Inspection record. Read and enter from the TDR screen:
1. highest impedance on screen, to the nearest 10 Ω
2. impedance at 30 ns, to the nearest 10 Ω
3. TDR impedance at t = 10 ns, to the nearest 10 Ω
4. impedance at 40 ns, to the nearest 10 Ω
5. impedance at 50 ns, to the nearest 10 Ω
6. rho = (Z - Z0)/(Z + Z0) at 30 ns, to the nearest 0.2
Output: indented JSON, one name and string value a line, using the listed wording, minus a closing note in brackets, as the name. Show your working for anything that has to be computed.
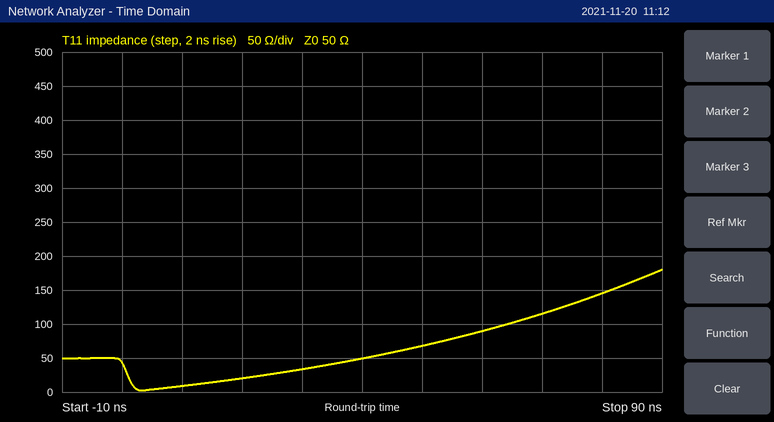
{
  "highest impedance on screen, to the nearest 10 Ω": "180 Ω",
  "impedance at 30 ns, to the nearest 10 Ω": "30 Ω",
  "TDR impedance at t = 10 ns, to the nearest 10 Ω": "10 Ω",
  "impedance at 40 ns, to the nearest 10 Ω": "50 Ω",
  "impedance at 50 ns, to the nearest 10 Ω": "70 Ω",
  "rho = (Z - Z0)/(Z + Z0) at 30 ns, to the nearest 0.2": "(30 − 50)/(30 + 50) ≈ -0.2"
}
